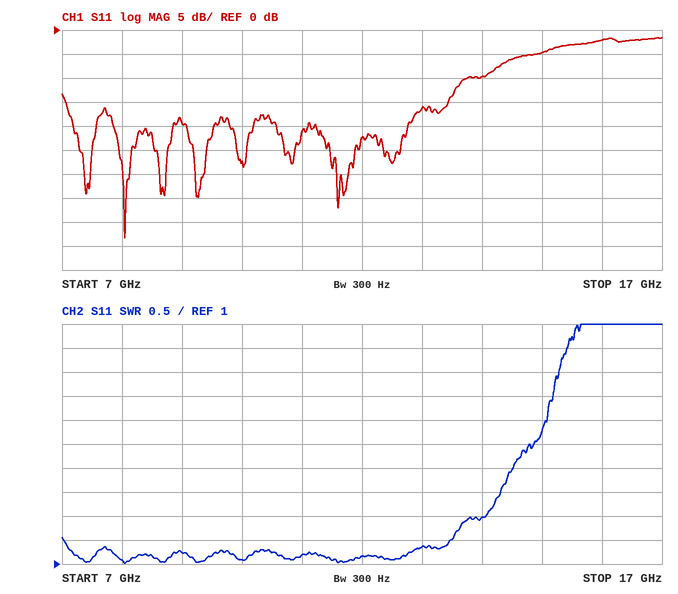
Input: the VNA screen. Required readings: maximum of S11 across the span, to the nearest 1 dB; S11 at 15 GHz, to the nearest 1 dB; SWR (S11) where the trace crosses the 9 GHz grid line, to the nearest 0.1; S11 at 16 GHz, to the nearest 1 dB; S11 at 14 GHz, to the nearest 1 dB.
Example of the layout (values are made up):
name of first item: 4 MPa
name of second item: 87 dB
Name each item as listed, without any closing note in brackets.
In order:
maximum of S11 across the span, to the nearest 1 dB: -2 dB
S11 at 15 GHz, to the nearest 1 dB: -5 dB
SWR (S11) where the trace crosses the 9 GHz grid line, to the nearest 0.1: 1.2
S11 at 16 GHz, to the nearest 1 dB: -2 dB
S11 at 14 GHz, to the nearest 1 dB: -10 dB
